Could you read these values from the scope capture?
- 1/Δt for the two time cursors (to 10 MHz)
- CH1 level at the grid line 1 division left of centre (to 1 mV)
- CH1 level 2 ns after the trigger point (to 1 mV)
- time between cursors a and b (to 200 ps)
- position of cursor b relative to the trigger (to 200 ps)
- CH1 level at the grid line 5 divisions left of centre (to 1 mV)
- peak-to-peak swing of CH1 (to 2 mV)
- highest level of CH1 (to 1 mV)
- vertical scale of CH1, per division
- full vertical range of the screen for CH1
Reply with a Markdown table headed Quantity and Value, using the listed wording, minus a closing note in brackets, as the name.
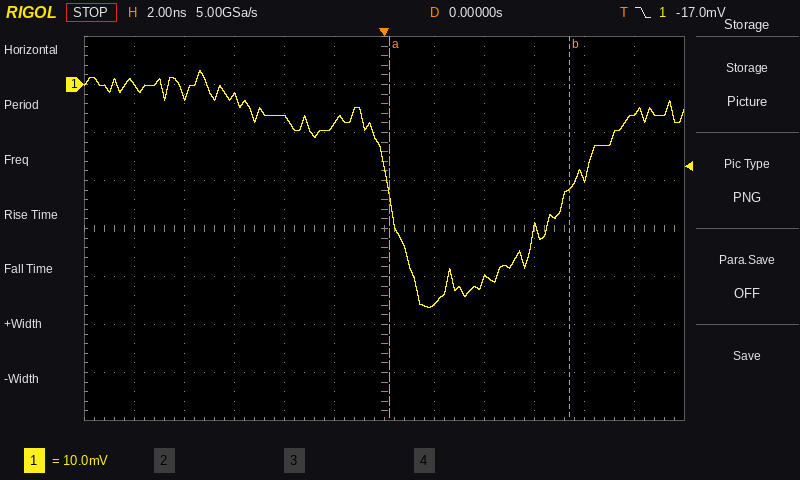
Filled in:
| Quantity | Value |
|---|---|
| 1/Δt for the two time cursors | 140 MHz |
| CH1 level at the grid line 1 division left of centre | -8 mV |
| CH1 level 2 ns after the trigger point | -46 mV |
| time between cursors a and b | 7.2 ns |
| position of cursor b relative to the trigger | +7.4 ns |
| CH1 level at the grid line 5 divisions left of centre | 0 mV |
| peak-to-peak swing of CH1 | 50 mV |
| highest level of CH1 | 3 mV |
| vertical scale of CH1, per division | 10 mV |
| full vertical range of the screen for CH1 | 80 mV |
